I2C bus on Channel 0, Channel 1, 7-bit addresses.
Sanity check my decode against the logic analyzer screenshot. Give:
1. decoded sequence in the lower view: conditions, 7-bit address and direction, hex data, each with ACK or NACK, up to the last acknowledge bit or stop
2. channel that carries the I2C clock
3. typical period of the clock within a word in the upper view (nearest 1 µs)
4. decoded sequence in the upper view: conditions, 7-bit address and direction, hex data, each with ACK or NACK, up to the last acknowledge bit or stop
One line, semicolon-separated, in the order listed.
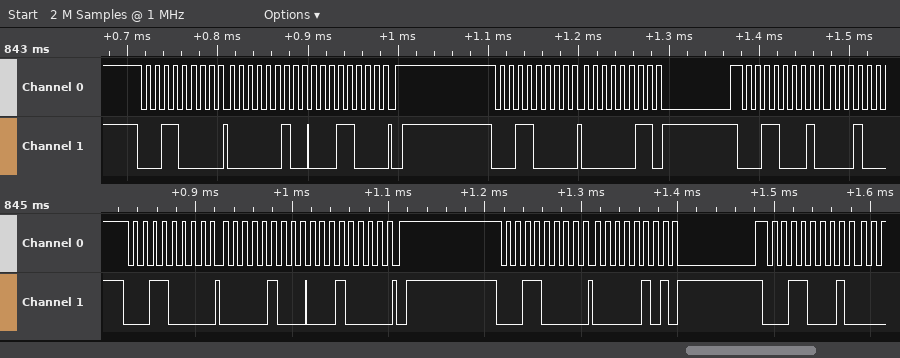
start, address 18 write ACK, 04 ACK, 10 ACK, stop, start, address 18 write ACK, 05 ACK, repeated start, address 18 read ACK; Channel 0; 10 µs; start, address 18 write ACK, 02 ACK, 18 ACK, stop, start, address 18 write ACK, 03 ACK, repeated start, address 18 read ACK
